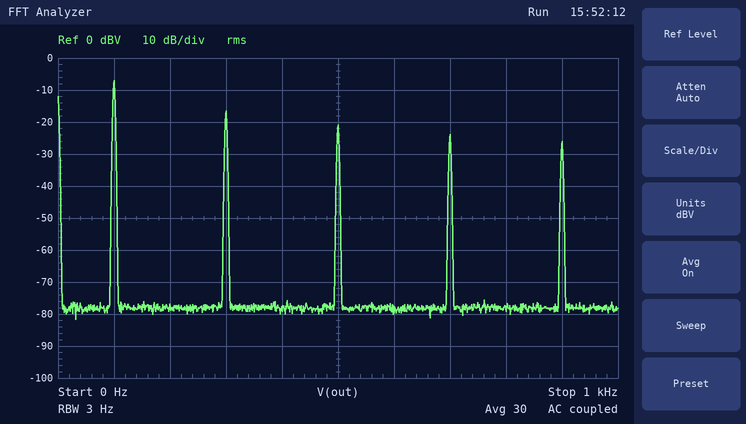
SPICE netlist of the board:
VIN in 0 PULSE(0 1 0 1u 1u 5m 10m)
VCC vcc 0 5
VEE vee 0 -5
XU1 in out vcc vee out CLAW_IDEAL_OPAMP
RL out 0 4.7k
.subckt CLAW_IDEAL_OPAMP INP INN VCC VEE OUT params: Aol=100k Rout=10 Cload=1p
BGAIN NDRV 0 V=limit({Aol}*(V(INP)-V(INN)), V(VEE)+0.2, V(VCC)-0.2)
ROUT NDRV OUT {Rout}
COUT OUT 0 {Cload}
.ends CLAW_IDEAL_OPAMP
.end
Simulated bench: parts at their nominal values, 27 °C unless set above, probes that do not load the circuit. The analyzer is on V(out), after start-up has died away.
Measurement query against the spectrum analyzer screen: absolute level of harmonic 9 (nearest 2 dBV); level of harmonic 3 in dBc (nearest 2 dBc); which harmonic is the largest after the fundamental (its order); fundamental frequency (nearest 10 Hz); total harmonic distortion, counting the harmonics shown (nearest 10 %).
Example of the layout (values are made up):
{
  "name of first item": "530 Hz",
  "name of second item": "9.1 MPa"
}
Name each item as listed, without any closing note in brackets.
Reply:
{
  "absolute level of harmonic 9": "-26 dBV",
  "level of harmonic 3 in dBc": "-10 dBc",
  "which harmonic is the largest after the fundamental": "3",
  "fundamental frequency": "100 Hz",
  "total harmonic distortion, counting the harmonics shown": "40 %"
}
